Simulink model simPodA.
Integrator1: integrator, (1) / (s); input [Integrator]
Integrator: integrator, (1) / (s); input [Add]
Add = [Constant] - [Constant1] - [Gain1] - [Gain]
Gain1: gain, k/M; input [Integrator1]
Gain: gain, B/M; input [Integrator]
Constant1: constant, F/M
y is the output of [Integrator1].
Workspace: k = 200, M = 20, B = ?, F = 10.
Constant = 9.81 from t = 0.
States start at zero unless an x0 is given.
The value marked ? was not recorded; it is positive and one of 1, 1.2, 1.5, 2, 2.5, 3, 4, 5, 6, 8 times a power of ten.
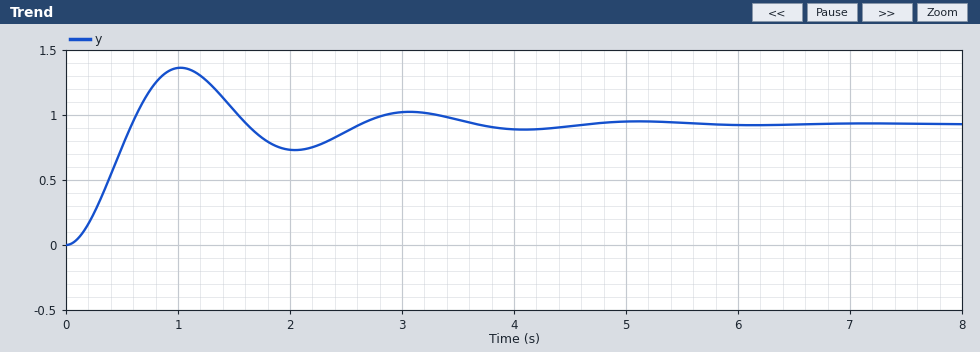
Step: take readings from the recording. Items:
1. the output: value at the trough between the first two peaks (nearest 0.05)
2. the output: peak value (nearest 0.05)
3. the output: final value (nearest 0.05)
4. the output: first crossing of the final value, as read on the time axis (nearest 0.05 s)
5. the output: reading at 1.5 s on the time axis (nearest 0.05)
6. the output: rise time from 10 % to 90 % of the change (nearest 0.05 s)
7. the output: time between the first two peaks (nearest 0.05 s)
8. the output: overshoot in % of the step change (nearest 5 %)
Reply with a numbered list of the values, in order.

1. 0.75
2. 1.35
3. 0.95
4. 0.60 s
5. 1.05
6. 0.40 s
7. 2.05 s
8. 45 %
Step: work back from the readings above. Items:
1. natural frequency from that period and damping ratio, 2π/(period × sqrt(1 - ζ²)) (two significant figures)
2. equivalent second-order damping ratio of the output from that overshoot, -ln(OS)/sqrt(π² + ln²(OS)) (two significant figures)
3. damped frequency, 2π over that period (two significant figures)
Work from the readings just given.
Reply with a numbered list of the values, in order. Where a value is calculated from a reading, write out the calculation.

1. 2π / (2.05 × sqrt(1 - 0.25²)) = 3.2 rad/s
2. ln(0.45) = -0.799; 0.799 / sqrt(9.870 + 0.638) = 0.25
3. 2π / 2.05 = 3.1 rad/s
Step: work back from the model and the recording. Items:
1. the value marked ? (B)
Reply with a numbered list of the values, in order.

1. 30
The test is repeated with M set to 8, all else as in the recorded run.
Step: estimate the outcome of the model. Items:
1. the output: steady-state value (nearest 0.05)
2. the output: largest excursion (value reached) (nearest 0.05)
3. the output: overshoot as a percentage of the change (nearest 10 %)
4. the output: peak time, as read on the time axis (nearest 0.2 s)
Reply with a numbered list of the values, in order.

1. 0.35
2. 0.45
3. 30 %
4. 0.6 s
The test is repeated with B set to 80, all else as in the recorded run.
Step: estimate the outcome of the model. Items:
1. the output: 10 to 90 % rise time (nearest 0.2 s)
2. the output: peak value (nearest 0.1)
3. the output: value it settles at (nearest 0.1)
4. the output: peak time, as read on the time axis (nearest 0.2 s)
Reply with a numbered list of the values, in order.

1. 0.6 s
2. 1.0
3. 0.9
4. 1.2 s
